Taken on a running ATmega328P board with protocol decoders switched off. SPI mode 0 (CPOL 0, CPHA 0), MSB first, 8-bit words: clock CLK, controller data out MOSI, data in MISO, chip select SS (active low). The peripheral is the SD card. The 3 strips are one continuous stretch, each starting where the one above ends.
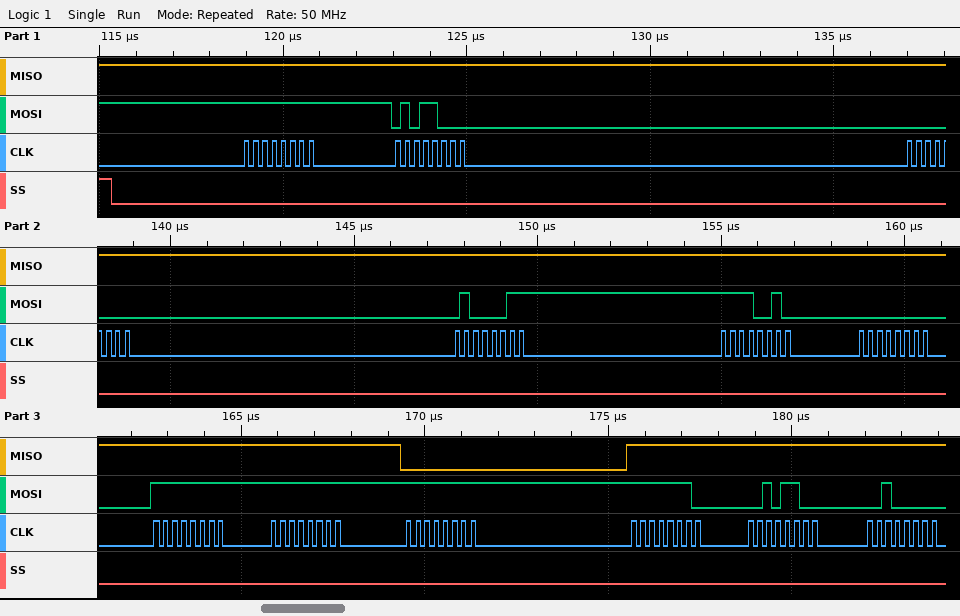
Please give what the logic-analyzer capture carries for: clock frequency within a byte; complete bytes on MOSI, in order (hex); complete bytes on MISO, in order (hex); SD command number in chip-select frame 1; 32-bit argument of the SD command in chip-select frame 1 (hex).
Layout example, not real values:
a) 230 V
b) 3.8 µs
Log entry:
a) 4 MHz
b) FF 58 00 43 F2 00 FF FF FF FE 2C 20
c) FF FF FF FF FF FF FF FF 00 FF FF FF
d) CMD24
e) 0x0043F200
